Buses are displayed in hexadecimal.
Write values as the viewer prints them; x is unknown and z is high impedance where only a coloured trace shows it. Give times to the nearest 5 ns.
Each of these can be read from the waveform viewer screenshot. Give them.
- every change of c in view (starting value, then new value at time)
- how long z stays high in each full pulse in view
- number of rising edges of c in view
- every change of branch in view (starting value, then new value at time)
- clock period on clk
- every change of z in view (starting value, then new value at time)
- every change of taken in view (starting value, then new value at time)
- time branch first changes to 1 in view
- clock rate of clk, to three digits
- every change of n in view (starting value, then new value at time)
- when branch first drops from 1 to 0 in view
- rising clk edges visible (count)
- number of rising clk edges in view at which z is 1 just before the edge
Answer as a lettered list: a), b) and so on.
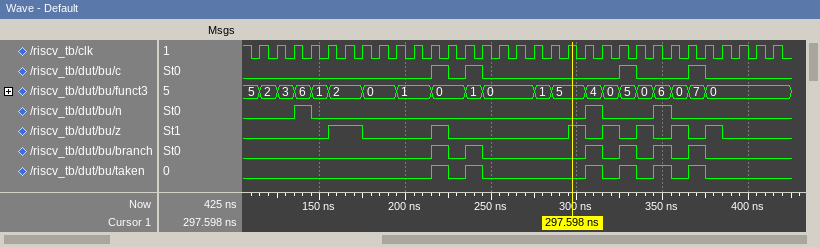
a) 0, 1 at 215 ns, 0 at 225 ns, 1 at 235 ns, 0 at 245 ns, 1 at 325 ns, 0 at 335 ns, 1 at 365 ns, 0 at 375 ns
b) 20 ns, 10 ns, 10 ns, 10 ns, 10 ns, 10 ns, 10 ns
c) 4
d) 0, 1 at 215 ns, 0 at 225 ns, 1 at 235 ns, 0 at 245 ns, 1 at 305 ns, 0 at 315 ns, 1 at 325 ns, 0 at 335 ns, 1 at 345 ns, 0 at 355 ns, 1 at 365 ns, 0 at 375 ns
e) 10 ns
f) 0, 1 at 155 ns, 0 at 175 ns, 1 at 215 ns, 0 at 225 ns, 1 at 295 ns, 0 at 305 ns, 1 at 315 ns, 0 at 325 ns, 1 at 335 ns, 0 at 345 ns, 1 at 355 ns, 0 at 365 ns, 1 at 375 ns, 0 at 385 ns
g) 0, 1 at 215 ns, 0 at 225 ns, 1 at 235 ns, 0 at 245 ns, 1 at 305 ns, 0 at 315 ns, 1 at 325 ns, 0 at 335 ns, 1 at 345 ns, 0 at 355 ns, 1 at 365 ns, 0 at 375 ns
h) 215 ns
i) 100 MHz
j) 0, 1 at 135 ns, 0 at 145 ns, 1 at 305 ns, 0 at 315 ns, 1 at 345 ns, 0 at 355 ns
k) 225 ns
l) 31
m) 8
